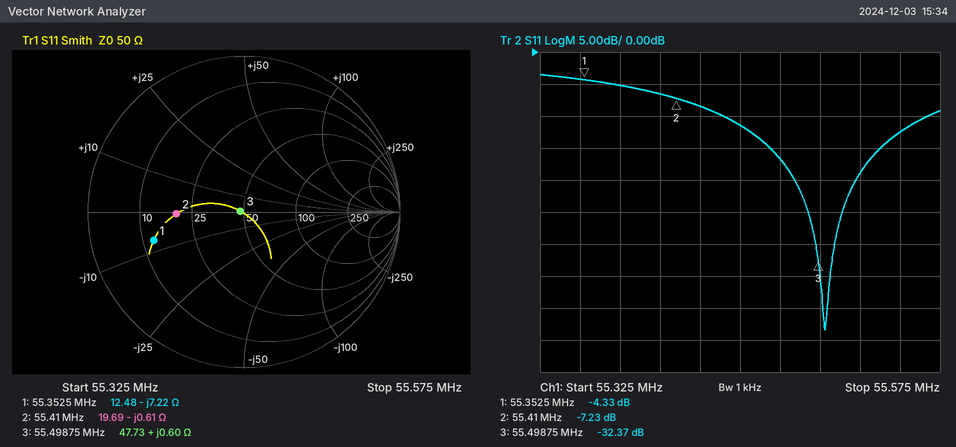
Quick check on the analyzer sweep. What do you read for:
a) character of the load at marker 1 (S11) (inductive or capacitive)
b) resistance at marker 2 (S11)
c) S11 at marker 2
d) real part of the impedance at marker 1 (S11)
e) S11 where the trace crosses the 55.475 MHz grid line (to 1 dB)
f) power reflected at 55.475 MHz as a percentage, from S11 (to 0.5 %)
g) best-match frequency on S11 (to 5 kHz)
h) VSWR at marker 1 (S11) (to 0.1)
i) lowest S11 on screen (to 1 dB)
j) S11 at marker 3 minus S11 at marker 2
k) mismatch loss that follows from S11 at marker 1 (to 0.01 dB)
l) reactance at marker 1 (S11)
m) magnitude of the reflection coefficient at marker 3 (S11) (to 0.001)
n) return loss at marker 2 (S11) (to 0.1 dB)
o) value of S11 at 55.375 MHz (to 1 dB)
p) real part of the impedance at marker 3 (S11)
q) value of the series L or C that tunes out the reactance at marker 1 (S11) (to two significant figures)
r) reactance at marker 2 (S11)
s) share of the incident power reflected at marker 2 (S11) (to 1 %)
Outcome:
capacitive
19.69 Ω
-7.23 dB
12.48 Ω
-17 dB
2.0 %
55.505 MHz
4.1
-43 dB
-25.14 dB
2.00 dB
-7.22 Ω
0.024
7.2 dB
-5 dB
47.73 Ω
21 nH
-0.61 Ω
19 %
